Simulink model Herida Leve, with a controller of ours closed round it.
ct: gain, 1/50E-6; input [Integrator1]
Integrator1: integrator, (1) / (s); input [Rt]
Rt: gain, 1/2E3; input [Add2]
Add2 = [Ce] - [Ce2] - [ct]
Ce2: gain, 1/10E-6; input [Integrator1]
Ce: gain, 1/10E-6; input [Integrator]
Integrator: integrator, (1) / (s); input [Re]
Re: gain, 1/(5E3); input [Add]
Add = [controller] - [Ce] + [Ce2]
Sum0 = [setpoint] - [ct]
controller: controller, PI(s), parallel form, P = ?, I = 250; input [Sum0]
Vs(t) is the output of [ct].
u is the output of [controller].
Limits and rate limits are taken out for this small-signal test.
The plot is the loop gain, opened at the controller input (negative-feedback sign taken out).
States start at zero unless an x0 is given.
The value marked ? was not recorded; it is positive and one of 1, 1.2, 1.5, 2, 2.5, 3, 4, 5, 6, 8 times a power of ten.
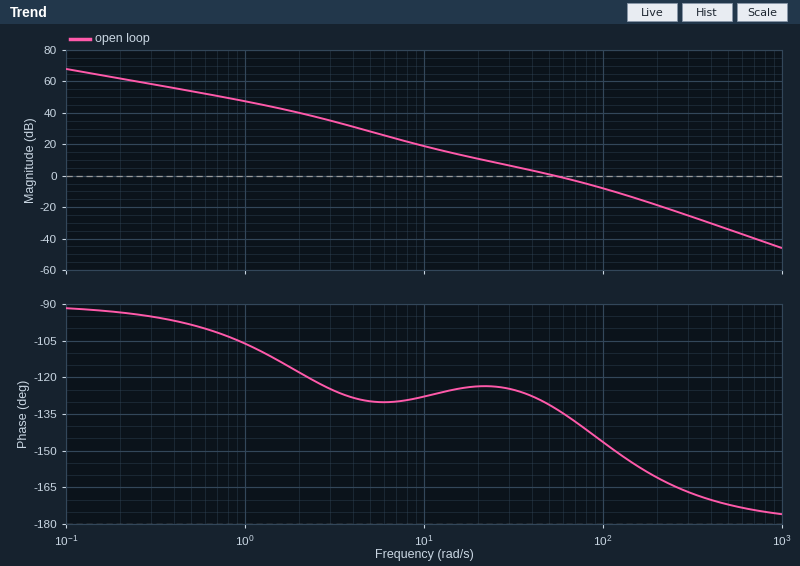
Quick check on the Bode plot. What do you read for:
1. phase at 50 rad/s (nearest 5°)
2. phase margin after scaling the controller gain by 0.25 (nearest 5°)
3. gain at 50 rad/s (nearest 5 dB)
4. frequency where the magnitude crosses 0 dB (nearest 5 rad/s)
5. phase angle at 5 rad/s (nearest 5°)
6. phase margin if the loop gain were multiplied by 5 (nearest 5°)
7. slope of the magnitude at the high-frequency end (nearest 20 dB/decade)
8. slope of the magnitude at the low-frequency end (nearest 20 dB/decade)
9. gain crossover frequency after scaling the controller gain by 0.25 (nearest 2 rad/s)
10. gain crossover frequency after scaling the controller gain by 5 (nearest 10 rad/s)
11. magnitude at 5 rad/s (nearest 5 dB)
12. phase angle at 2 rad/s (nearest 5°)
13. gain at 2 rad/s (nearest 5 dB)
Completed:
-130°
55°
0 dB
55 rad/s
-130°
25°
-40 dB/decade
-20 dB/decade
18 rad/s
150 rad/s
30 dB
-120°
40 dB
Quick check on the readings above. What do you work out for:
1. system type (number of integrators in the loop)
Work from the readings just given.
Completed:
1
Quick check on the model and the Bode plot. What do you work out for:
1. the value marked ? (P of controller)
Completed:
25
